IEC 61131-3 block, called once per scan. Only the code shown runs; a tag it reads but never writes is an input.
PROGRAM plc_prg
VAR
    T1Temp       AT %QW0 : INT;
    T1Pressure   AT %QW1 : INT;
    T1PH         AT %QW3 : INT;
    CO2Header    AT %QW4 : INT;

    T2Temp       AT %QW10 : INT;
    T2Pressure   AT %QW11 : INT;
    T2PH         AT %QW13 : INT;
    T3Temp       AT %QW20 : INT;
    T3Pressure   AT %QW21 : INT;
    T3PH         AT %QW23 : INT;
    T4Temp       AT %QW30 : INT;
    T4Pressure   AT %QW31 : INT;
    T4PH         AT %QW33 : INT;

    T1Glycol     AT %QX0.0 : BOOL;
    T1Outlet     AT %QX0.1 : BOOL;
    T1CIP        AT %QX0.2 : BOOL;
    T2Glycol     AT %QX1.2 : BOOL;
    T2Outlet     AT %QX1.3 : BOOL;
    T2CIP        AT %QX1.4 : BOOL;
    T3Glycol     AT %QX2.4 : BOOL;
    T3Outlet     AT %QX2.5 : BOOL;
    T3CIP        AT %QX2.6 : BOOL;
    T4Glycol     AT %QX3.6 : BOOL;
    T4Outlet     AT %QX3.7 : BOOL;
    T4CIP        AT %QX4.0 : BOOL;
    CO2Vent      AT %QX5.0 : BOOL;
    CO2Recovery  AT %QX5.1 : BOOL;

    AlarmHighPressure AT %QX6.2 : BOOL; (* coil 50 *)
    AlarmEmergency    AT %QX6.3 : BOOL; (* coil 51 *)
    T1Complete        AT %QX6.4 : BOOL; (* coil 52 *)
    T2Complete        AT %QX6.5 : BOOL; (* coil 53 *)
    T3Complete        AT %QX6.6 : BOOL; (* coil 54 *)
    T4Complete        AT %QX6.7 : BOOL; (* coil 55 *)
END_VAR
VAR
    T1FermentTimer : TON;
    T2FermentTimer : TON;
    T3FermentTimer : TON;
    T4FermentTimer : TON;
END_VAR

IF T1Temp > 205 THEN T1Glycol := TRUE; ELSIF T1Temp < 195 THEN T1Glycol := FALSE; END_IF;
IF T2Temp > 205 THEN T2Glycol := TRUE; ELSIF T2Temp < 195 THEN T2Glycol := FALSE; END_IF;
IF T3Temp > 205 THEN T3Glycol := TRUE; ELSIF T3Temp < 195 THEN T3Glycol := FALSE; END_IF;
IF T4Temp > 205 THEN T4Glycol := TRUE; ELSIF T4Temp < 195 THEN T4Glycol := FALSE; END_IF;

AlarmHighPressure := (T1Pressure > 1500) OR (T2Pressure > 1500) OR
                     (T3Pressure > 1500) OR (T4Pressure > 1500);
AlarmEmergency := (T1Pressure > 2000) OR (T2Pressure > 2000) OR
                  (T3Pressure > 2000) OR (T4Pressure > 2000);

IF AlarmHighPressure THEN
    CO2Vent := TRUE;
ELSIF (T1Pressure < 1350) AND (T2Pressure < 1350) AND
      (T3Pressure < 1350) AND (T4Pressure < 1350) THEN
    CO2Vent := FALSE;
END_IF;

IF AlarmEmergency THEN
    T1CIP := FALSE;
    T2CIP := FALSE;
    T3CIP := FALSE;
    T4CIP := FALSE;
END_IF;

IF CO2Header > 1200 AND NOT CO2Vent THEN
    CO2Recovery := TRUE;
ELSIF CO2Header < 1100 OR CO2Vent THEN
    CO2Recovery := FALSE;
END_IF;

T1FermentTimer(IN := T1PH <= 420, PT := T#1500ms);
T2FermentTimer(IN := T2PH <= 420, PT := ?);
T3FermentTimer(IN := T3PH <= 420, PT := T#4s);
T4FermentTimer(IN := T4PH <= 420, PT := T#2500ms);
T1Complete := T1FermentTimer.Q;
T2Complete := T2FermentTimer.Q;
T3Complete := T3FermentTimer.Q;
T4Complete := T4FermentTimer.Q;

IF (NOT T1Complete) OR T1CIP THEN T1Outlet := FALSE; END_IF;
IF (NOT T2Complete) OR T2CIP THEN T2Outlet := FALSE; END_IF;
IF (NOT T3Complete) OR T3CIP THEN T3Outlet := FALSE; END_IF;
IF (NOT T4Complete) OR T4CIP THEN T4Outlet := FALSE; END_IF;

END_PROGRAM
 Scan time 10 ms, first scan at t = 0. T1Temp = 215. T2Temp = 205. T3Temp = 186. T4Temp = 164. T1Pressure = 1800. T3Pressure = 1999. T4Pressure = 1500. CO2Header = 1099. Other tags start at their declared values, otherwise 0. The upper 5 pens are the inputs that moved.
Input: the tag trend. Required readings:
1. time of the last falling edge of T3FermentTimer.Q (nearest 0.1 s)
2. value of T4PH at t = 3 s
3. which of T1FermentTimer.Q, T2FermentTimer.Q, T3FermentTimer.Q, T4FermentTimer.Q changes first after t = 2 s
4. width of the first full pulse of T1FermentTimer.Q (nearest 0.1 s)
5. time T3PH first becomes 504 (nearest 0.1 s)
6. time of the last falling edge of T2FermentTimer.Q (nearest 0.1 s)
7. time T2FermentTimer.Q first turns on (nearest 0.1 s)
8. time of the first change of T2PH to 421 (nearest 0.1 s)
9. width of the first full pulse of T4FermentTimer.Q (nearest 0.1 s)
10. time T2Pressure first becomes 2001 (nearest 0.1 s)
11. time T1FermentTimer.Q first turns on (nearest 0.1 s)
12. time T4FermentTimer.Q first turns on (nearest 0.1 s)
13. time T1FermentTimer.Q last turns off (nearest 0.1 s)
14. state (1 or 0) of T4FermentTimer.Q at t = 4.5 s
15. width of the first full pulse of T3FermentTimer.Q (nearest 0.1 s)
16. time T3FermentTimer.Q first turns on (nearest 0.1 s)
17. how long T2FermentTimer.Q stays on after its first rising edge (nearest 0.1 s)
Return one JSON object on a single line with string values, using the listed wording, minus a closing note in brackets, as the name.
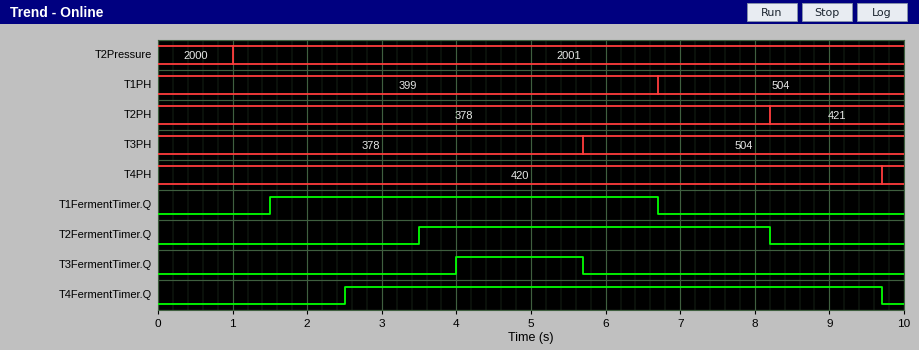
{"time of the last falling edge of T3FermentTimer.Q": "5.7 s", "value of T4PH at t = 3 s": "420", "which of T1FermentTimer.Q, T2FermentTimer.Q, T3FermentTimer.Q, T4FermentTimer.Q changes first after t = 2 s": "T4FermentTimer.Q", "width of the first full pulse of T1FermentTimer.Q": "5.2 s", "time T3PH first becomes 504": "5.7 s", "time of the last falling edge of T2FermentTimer.Q": "8.2 s", "time T2FermentTimer.Q first turns on": "3.5 s", "time of the first change of T2PH to 421": "8.2 s", "width of the first full pulse of T4FermentTimer.Q": "7.2 s", "time T2Pressure first becomes 2001": "1.0 s", "time T1FermentTimer.Q first turns on": "1.5 s", "time T4FermentTimer.Q first turns on": "2.5 s", "time T1FermentTimer.Q last turns off": "6.7 s", "state (1 or 0) of T4FermentTimer.Q at t = 4.5 s": "1", "width of the first full pulse of T3FermentTimer.Q": "1.7 s", "time T3FermentTimer.Q first turns on": "4.0 s", "how long T2FermentTimer.Q stays on after its first rising edge": "4.7 s"}
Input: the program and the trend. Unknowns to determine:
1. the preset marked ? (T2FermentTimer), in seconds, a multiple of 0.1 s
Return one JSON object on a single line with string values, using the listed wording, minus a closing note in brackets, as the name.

{"the preset marked ? (T2FermentTimer), in seconds, a multiple of 0.1 s": "3.5 s"}
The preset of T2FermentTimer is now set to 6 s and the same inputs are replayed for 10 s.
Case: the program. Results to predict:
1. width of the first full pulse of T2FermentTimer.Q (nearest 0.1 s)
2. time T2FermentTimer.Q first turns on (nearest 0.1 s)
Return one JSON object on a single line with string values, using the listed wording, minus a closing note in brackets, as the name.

{"width of the first full pulse of T2FermentTimer.Q": "2.2 s", "time T2FermentTimer.Q first turns on": "6.0 s"}
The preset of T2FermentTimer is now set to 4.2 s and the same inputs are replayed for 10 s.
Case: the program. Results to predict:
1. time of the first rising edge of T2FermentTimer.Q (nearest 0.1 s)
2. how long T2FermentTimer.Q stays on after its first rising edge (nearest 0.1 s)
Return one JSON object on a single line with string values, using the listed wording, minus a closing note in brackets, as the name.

{"time of the first rising edge of T2FermentTimer.Q": "4.2 s", "how long T2FermentTimer.Q stays on after its first rising edge": "4.0 s"}
